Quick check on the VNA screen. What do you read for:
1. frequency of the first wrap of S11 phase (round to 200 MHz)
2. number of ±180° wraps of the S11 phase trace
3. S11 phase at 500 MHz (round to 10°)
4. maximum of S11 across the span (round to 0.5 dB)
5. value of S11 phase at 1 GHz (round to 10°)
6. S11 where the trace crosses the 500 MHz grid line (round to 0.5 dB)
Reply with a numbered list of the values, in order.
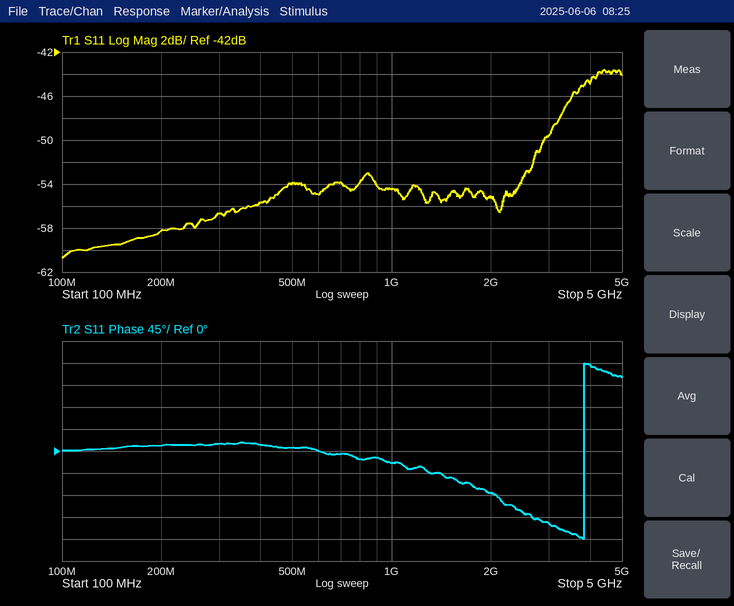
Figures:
1. 3.8 GHz
2. 1
3. 10°
4. -43.5 dB
5. -20°
6. -54.0 dB
